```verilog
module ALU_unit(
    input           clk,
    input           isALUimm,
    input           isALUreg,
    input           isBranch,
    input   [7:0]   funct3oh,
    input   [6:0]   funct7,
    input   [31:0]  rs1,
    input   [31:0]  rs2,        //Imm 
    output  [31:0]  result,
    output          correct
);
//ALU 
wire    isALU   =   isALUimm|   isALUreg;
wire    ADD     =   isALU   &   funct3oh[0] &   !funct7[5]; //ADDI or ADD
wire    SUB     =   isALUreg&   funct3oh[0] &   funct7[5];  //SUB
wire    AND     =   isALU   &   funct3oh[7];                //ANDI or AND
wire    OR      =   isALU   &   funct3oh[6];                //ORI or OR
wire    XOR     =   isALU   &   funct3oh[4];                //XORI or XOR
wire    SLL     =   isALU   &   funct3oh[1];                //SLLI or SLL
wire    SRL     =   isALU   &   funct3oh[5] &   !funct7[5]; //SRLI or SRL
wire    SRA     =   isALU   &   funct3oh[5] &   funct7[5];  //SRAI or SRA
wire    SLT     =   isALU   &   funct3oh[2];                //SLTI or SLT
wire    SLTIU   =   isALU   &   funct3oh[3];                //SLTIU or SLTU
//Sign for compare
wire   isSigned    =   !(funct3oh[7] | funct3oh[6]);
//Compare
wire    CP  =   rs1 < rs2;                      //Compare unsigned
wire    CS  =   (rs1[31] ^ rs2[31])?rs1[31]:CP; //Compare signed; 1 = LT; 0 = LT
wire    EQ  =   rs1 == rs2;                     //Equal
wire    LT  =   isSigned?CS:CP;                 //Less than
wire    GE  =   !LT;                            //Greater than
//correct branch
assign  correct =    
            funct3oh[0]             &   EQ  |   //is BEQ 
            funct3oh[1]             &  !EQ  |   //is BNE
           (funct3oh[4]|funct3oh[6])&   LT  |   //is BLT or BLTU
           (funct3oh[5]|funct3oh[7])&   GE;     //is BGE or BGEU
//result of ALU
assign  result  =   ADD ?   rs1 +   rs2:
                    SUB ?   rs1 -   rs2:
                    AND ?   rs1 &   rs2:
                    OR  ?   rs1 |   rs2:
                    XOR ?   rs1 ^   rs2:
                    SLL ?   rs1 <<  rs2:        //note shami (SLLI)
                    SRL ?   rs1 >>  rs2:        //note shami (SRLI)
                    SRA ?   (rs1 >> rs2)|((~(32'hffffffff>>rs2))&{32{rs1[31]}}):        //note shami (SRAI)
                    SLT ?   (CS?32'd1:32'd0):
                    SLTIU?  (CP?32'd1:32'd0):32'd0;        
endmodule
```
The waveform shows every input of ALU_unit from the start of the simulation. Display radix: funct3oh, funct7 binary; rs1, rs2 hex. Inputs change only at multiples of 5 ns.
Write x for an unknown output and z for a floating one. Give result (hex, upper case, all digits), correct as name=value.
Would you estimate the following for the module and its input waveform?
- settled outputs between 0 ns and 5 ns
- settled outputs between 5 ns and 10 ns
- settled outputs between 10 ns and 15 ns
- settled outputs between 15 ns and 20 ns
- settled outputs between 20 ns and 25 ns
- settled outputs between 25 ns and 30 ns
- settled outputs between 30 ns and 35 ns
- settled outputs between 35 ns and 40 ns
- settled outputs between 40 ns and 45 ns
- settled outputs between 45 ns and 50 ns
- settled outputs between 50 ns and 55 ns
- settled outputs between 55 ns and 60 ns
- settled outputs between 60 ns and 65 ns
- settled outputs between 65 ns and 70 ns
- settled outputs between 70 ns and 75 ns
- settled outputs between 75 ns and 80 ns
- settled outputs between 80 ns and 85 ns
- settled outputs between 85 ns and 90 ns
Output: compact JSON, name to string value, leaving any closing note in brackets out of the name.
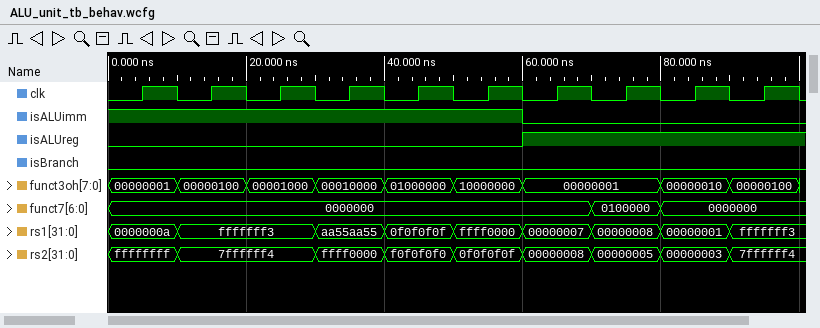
{"settled outputs between 0 ns and 5 ns": "result=00000009, correct=0", "settled outputs between 5 ns and 10 ns": "result=00000009, correct=0", "settled outputs between 10 ns and 15 ns": "result=00000001, correct=0", "settled outputs between 15 ns and 20 ns": "result=00000001, correct=0", "settled outputs between 20 ns and 25 ns": "result=00000000, correct=0", "settled outputs between 25 ns and 30 ns": "result=00000000, correct=0", "settled outputs between 30 ns and 35 ns": "result=55AAAA55, correct=1", "settled outputs between 35 ns and 40 ns": "result=55AAAA55, correct=1", "settled outputs between 40 ns and 45 ns": "result=FFFFFFFF, correct=1", "settled outputs between 45 ns and 50 ns": "result=FFFFFFFF, correct=1", "settled outputs between 50 ns and 55 ns": "result=0F0F0000, correct=1", "settled outputs between 55 ns and 60 ns": "result=0F0F0000, correct=1", "settled outputs between 60 ns and 65 ns": "result=0000000F, correct=0", "settled outputs between 65 ns and 70 ns": "result=0000000F, correct=0", "settled outputs between 70 ns and 75 ns": "result=00000003, correct=0", "settled outputs between 75 ns and 80 ns": "result=00000003, correct=0", "settled outputs between 80 ns and 85 ns": "result=00000008, correct=1", "settled outputs between 85 ns and 90 ns": "result=00000008, correct=1"}
